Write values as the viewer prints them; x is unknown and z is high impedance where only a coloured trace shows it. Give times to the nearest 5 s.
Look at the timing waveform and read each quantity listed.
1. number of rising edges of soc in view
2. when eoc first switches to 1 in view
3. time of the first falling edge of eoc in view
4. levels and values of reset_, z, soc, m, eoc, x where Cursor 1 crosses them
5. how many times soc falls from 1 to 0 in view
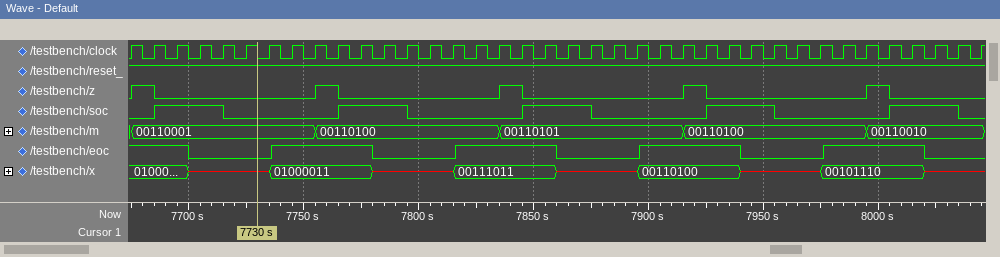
5
7735 s
7700 s
reset_=1, z=0, soc=0, m=00110001, eoc=0, x=x
5
